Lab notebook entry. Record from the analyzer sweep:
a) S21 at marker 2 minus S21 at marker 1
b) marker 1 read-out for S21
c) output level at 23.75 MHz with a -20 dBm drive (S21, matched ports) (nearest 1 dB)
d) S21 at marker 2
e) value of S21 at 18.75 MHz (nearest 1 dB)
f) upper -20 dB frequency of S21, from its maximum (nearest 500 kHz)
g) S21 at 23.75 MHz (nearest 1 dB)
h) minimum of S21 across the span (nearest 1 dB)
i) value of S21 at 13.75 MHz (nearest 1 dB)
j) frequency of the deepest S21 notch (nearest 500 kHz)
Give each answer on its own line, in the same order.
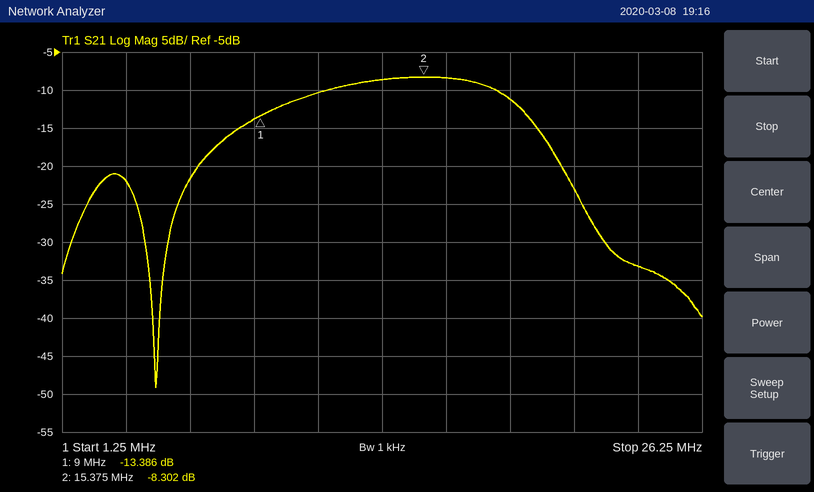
5.084 dB
-13.386 dB
-53 dBm
-8.302 dB
-11 dB
22.0 MHz
-33 dB
-49 dB
-9 dB
5.0 MHz
